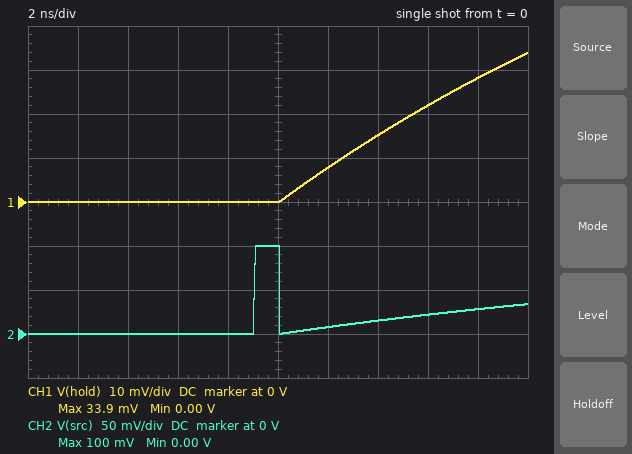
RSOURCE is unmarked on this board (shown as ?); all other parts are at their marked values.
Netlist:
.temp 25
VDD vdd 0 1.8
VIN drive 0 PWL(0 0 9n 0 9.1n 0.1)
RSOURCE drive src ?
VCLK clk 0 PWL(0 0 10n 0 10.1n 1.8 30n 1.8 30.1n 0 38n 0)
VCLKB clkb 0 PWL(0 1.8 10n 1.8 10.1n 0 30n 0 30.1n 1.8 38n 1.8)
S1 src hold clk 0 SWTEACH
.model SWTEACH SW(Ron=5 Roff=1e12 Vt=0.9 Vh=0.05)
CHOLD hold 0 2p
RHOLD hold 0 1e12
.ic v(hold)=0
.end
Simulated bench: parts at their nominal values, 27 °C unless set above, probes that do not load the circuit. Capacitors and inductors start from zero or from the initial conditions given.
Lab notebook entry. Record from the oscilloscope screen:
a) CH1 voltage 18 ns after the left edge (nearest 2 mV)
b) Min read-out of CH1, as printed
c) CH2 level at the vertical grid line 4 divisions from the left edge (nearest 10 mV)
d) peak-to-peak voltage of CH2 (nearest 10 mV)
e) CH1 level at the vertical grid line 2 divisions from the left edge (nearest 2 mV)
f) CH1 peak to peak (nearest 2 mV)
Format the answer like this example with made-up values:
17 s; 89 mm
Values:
28 mV; 0.00 V; 0 V; 100 mV; 0 V; 34 mV
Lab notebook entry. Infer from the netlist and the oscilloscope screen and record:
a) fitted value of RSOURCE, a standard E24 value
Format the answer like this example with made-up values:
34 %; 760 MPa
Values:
12 kΩ
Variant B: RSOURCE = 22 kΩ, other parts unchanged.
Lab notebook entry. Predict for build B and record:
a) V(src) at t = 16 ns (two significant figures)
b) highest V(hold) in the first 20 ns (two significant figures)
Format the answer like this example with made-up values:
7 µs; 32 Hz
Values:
13 mV; 20 mV
